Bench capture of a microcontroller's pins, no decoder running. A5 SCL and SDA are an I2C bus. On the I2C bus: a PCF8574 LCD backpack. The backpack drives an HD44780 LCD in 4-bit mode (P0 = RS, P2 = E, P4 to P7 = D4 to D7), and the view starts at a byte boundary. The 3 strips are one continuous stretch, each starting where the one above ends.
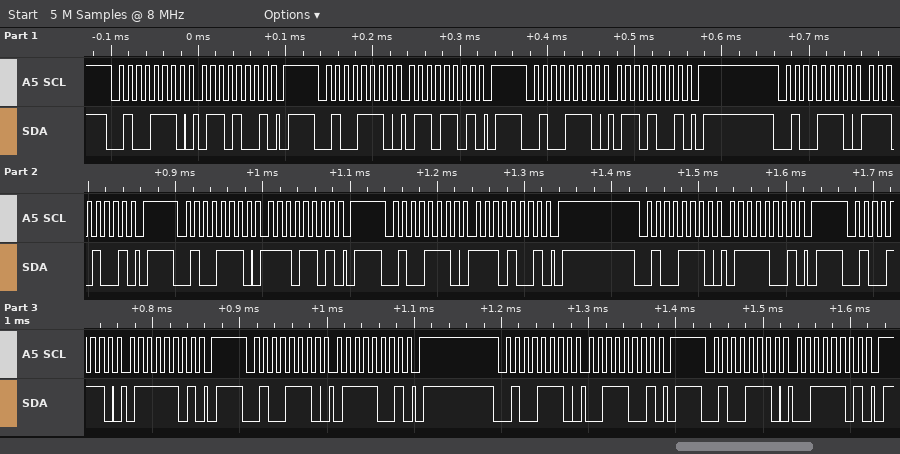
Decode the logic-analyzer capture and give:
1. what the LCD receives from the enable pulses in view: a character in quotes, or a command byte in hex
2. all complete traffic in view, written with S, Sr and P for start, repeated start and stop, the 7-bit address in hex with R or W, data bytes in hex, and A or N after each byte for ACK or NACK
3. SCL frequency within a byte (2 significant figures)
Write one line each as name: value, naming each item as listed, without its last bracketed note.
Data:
what the LCD receives from the enable pulses in view: a character in quotes, or a command byte in hex: 'n'
all complete traffic in view, written with S, Sr and P for start, repeated start and stop, the 7-bit address in hex with R or W, data bytes in hex, and A or N after each byte for ACK or NACK: S 27W A 69 A P S 27W A 6D A P S 27W A 69 A P S 27W A E9 A P S 27W A ED A P S 27W A E9 A P S 27W A 79 A P S 27W A 7D A P S 27W A 79 A P S 27W A 39 A P S 27W A 3D A P
SCL frequency within a byte: 100 kHz
